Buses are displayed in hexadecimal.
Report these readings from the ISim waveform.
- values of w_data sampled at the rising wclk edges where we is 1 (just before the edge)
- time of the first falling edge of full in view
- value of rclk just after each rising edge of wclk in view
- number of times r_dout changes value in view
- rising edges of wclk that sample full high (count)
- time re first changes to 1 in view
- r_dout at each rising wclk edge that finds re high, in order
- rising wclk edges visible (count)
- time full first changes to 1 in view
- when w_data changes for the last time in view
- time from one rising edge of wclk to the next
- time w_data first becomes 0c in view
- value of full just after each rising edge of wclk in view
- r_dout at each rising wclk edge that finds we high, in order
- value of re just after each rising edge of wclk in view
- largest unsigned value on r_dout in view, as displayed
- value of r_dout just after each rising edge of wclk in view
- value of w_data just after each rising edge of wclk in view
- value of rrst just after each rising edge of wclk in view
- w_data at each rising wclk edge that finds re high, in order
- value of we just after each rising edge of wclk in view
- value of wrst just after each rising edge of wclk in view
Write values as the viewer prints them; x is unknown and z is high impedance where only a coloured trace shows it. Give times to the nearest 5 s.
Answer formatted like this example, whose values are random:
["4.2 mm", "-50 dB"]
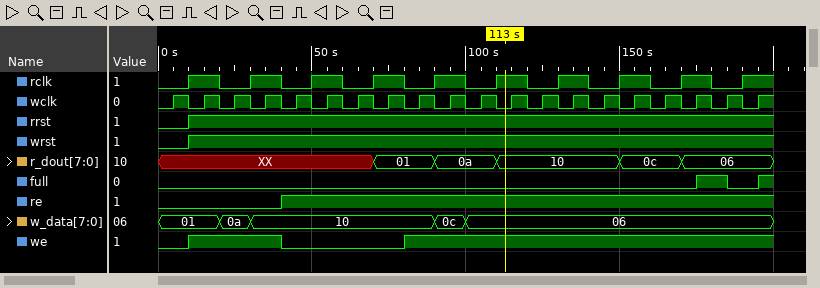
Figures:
["01, 0a, 10, 10, 0c, 06, 06, 06, 06, 06, 06, 06, 06, 06, 06", "185 s", "0 1 0 1 0 1 0 1 0 1 0 1 0 1 0 1 0 1 0 1", "5", "1", "40 s", "XX, XX, XX, 01, 01, 0a, 0a, 10, 10, 10, 10, 0c, 0c, 06, 06, 06", "20", "175 s", "100 s", "10 s", "90 s", "0 0 0 0 0 0 0 0 0 0 0 0 0 0 0 0 0 1 0 1", "XX, XX, XX, 01, 0a, 0a, 10, 10, 10, 10, 0c, 0c, 06, 06, 06", "0 0 0 0 1 1 1 1 1 1 1 1 1 1 1 1 1 1 1 1", "10", "XX, XX, XX, XX, XX, XX, XX, 01, 01, 0a, 0a, 10, 10, 10, 10, 0c, 0c, 06, 06, 06", "01, 01, 0a, 10, 10, 10, 10, 10, 10, 0c, 06, 06, 06, 06, 06, 06, 06, 06, 06, 06", "0 1 1 1 1 1 1 1 1 1 1 1 1 1 1 1 1 1 1 1", "10, 10, 10, 10, 10, 0c, 06, 06, 06, 06, 06, 06, 06, 06, 06, 06", "0 1 1 1 0 0 0 0 1 1 1 1 1 1 1 1 1 1 1 1", "0 1 1 1 1 1 1 1 1 1 1 1 1 1 1 1 1 1 1 1"]
